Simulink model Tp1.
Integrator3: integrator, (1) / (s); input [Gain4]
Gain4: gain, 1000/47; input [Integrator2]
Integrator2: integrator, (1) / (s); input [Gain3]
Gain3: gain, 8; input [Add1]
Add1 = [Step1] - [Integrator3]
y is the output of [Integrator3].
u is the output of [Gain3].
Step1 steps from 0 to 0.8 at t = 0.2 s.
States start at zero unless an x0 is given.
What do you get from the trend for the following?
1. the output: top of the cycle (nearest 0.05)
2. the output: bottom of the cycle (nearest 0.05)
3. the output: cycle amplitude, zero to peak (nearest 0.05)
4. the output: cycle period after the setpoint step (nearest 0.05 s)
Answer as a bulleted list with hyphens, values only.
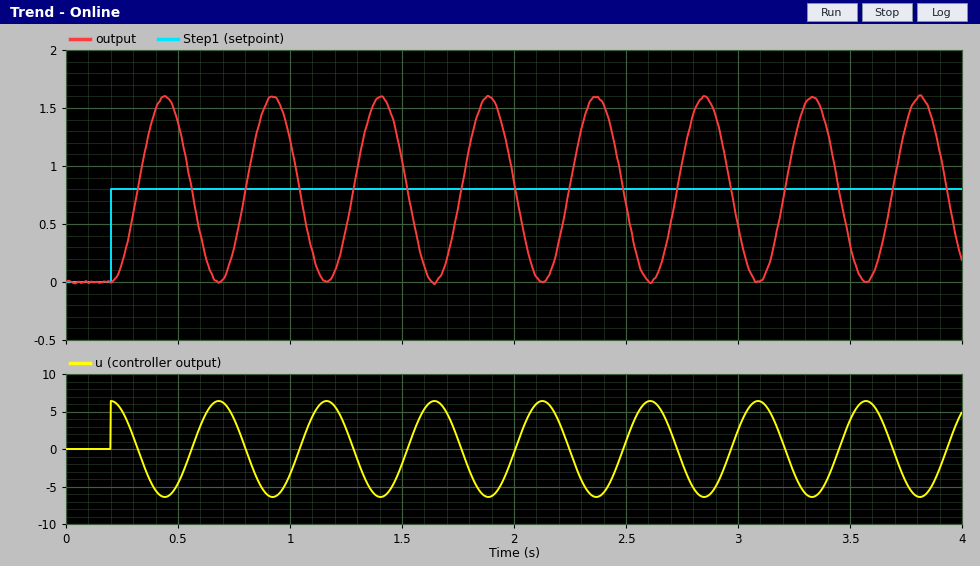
- 1.60
- 0.00
- 0.80
- 0.50 s
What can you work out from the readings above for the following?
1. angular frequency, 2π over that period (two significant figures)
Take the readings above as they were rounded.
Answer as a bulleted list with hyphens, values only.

- 13 rad/s
